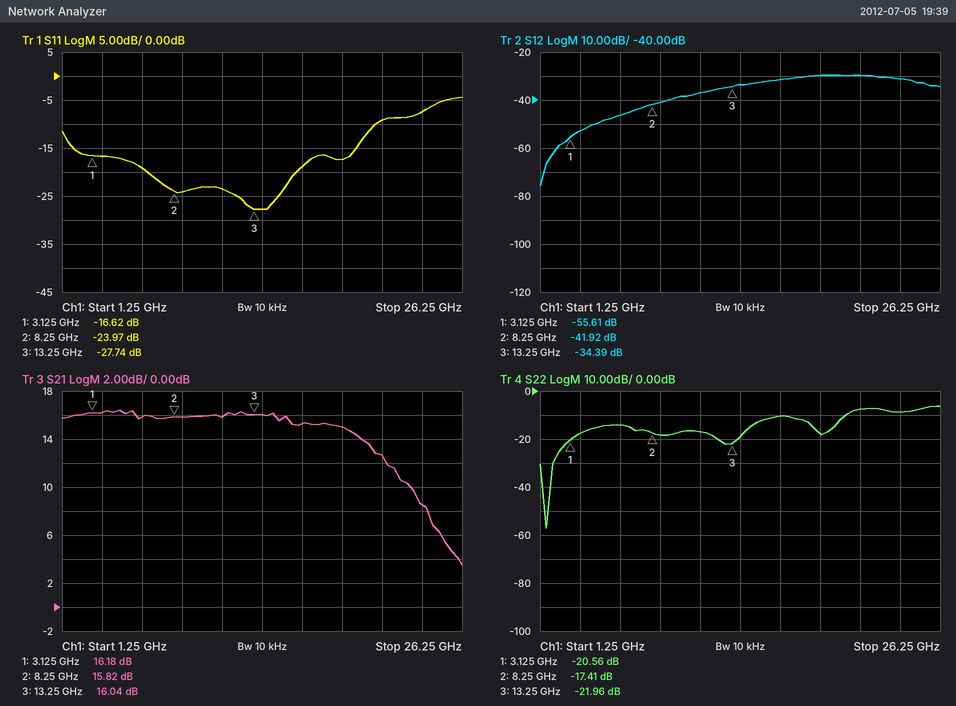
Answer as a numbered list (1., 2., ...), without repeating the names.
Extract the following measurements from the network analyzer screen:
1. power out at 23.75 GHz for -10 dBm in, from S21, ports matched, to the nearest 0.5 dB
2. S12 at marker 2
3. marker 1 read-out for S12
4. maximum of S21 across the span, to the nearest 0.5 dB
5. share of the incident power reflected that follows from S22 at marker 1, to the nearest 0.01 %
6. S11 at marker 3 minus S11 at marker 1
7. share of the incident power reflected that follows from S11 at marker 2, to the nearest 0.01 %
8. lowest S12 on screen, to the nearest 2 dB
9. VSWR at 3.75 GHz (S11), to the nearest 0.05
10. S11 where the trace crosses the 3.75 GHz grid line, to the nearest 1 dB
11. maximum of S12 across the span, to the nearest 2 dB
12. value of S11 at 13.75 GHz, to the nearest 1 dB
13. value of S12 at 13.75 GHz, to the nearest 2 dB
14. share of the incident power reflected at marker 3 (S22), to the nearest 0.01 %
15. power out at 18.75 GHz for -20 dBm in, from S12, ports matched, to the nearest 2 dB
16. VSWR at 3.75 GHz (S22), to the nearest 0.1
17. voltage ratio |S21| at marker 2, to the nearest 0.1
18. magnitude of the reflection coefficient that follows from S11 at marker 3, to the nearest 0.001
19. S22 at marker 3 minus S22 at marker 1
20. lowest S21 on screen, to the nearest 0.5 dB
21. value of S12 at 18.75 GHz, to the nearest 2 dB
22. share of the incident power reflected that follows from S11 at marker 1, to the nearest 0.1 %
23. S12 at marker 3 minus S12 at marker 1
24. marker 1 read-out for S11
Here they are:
1. -1.5 dBm
2. -41.92 dB
3. -55.61 dB
4. 16.5 dB
5. 0.88 %
6. -11.12 dB
7. 0.40 %
8. -76 dB
9. 1.35
10. -17 dB
11. -30 dB
12. -28 dB
13. -34 dB
14. 0.64 %
15. -50 dBm
16. 1.3
17. 6.2
18. 0.041
19. -1.40 dB
20. 3.5 dB
21. -30 dB
22. 2.2 %
23. 21.22 dB
24. -16.62 dB
